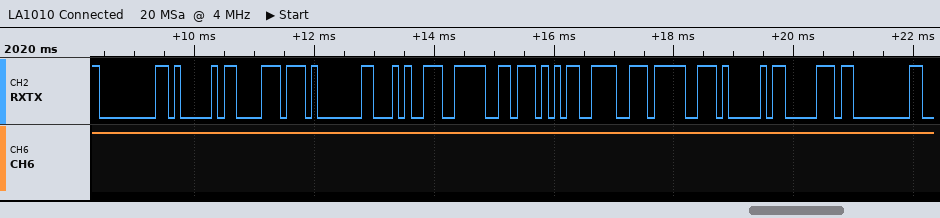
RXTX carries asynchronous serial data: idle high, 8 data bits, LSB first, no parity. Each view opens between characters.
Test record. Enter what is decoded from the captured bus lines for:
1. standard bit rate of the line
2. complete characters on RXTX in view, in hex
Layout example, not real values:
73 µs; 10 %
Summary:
9600 baud; 00, 41, B8, 01, 94, 3E, 57, 9E, 9F, 41, 70, 00
